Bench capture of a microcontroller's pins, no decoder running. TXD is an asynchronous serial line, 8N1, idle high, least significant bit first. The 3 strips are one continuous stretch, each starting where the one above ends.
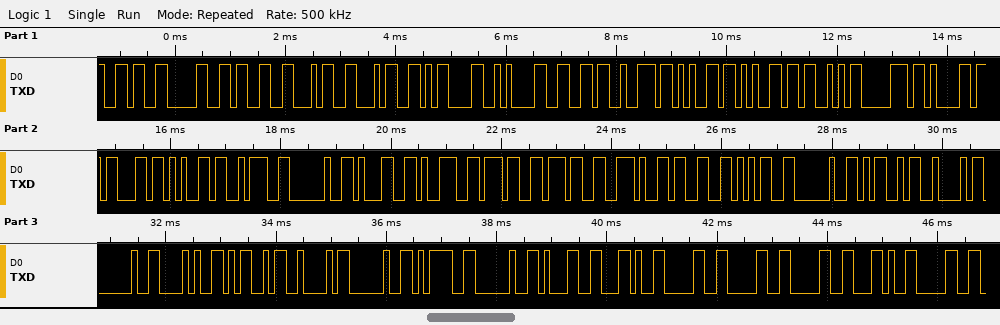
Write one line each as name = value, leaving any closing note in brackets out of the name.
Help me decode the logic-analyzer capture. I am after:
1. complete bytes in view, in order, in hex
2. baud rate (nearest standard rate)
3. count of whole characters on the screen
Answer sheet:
complete bytes in view, in order, in hex = 36 30 33 34 34 0D 0A 66 72 65 65 53 70 61 63 65 3A 20 31 39 37 37 2E 33 35 20 4D 42 20 28 4D 42 20 3D 20 31 2C 30 30 30 2C 30
baud rate = 9600 baud
count of whole characters on the screen = 42
